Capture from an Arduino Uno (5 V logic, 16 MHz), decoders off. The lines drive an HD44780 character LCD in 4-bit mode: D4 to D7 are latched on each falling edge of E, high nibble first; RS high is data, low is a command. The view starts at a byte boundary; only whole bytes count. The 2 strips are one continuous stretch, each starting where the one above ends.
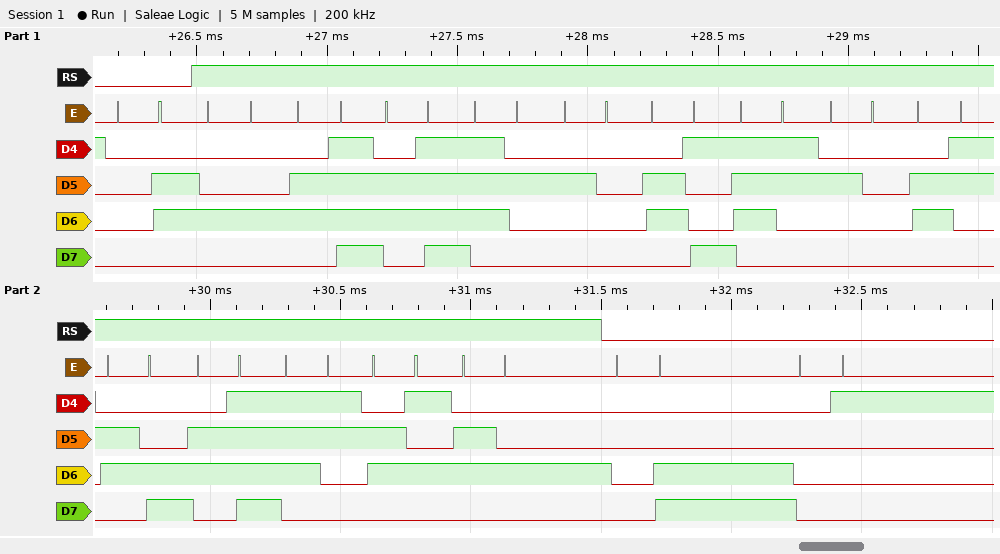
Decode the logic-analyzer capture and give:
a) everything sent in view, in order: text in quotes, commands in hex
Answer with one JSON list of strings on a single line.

["0x06 \"Door is closed\" 0x0C 0x01"]
